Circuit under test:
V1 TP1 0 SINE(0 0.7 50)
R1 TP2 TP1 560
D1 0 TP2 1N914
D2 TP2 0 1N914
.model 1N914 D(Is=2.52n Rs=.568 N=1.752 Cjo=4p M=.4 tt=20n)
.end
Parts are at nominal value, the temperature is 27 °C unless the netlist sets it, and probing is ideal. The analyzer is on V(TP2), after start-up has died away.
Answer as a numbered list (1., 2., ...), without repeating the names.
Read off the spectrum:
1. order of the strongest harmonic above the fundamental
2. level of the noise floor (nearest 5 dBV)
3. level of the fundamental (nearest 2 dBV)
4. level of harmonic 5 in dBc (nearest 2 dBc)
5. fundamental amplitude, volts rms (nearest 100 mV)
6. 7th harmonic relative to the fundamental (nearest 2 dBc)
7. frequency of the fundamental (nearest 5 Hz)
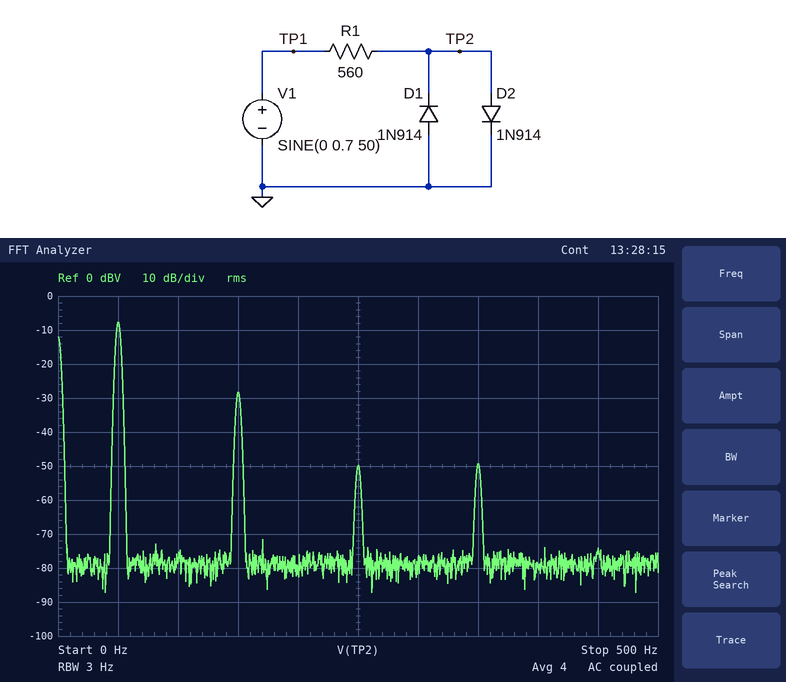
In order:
1. 3
2. -80 dBV
3. -8 dBV
4. -42 dBc
5. 400 mV
6. -42 dBc
7. 50 Hz
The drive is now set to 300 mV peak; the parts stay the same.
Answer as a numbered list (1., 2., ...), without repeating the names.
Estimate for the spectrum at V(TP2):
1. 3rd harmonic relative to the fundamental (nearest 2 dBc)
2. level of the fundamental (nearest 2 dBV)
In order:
1. -60 dBc
2. -14 dBV
